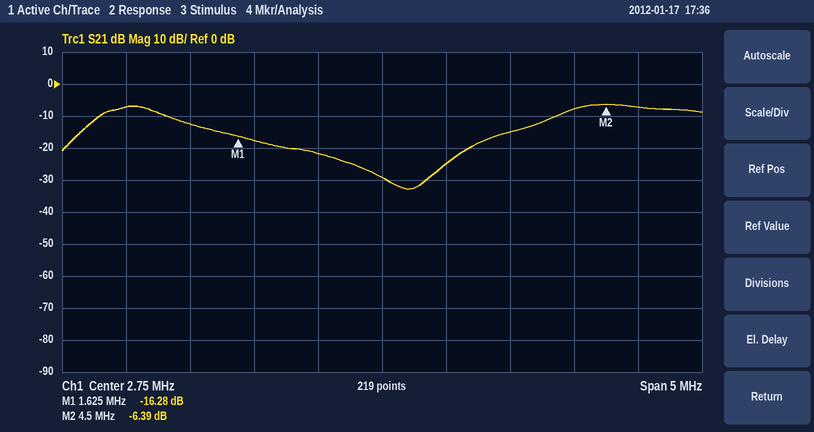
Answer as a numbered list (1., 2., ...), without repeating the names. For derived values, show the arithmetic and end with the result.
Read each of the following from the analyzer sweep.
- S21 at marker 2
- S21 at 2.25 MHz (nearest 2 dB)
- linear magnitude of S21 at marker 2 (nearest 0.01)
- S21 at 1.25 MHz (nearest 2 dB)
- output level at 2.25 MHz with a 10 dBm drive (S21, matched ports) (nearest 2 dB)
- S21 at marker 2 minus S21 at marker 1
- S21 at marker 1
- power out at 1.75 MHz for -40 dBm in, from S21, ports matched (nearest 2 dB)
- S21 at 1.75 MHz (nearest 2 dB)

1. -6.39 dB
2. -22 dB
3. 10^(-6.39/20) ≈ 0.48
4. -12 dB
5. 10 dBm + (-22 dB) = -12 dBm
6. -6.39 − (-16.28) = 9.89 dB
7. -16.28 dB
8. -40 dBm + (-18 dB) = -58 dBm
9. -18 dB
